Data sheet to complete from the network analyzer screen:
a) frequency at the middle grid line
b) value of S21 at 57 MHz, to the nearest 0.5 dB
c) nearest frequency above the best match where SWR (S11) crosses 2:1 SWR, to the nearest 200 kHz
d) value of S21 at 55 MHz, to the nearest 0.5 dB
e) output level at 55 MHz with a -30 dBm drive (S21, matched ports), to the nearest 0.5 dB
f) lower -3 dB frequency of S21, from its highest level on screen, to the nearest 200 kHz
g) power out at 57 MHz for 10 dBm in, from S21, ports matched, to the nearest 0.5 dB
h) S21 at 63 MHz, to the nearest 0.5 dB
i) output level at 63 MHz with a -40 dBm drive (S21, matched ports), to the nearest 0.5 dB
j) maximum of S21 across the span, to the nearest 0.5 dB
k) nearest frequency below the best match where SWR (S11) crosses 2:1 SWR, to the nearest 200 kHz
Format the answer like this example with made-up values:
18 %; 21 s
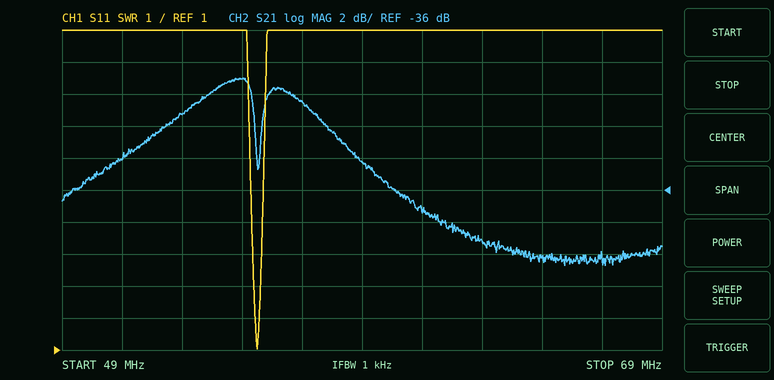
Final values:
59 MHz; -30.5 dB; 55.6 MHz; -29.0 dB; -59.0 dBm; 52.4 MHz; -20.5 dBm; -39.0 dB; -79.0 dBm; -29.0 dB; 55.4 MHz
